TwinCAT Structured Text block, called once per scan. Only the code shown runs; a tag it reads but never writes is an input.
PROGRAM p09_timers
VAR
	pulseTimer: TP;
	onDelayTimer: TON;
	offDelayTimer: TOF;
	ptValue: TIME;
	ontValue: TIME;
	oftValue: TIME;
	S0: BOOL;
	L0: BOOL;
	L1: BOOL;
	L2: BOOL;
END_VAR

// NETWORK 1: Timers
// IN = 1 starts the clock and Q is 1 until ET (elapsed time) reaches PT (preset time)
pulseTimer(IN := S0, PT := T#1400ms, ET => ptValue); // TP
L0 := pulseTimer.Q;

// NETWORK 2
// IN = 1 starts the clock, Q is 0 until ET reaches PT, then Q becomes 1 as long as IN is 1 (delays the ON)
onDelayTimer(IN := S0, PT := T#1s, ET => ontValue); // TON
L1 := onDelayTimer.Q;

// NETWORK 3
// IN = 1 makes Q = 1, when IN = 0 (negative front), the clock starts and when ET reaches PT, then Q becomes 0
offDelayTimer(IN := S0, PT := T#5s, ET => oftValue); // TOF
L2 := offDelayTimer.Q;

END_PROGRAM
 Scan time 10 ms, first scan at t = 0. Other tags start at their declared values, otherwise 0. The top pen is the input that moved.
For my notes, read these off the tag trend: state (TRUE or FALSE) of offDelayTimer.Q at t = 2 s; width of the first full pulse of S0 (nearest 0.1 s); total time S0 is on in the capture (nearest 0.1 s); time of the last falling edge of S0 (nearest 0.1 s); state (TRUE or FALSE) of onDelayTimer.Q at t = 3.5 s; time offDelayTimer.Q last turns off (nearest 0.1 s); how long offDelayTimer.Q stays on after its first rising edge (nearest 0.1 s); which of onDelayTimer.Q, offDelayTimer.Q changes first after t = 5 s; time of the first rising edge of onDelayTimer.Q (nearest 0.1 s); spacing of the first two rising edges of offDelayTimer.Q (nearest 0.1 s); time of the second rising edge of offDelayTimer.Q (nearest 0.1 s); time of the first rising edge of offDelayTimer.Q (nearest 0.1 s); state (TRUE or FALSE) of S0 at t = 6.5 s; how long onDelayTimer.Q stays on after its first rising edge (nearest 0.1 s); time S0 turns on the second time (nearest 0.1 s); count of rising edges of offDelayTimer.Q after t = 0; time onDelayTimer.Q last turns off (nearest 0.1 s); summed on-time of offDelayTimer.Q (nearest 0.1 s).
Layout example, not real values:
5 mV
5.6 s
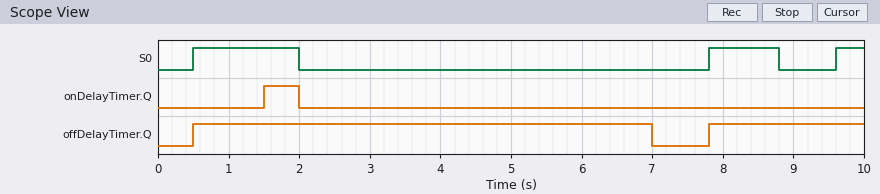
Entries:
TRUE
1.5 s
2.9 s
8.8 s
FALSE
7.0 s
6.5 s
offDelayTimer.Q
1.5 s
7.3 s
7.8 s
0.5 s
FALSE
0.5 s
7.8 s
2
2.0 s
8.7 s
